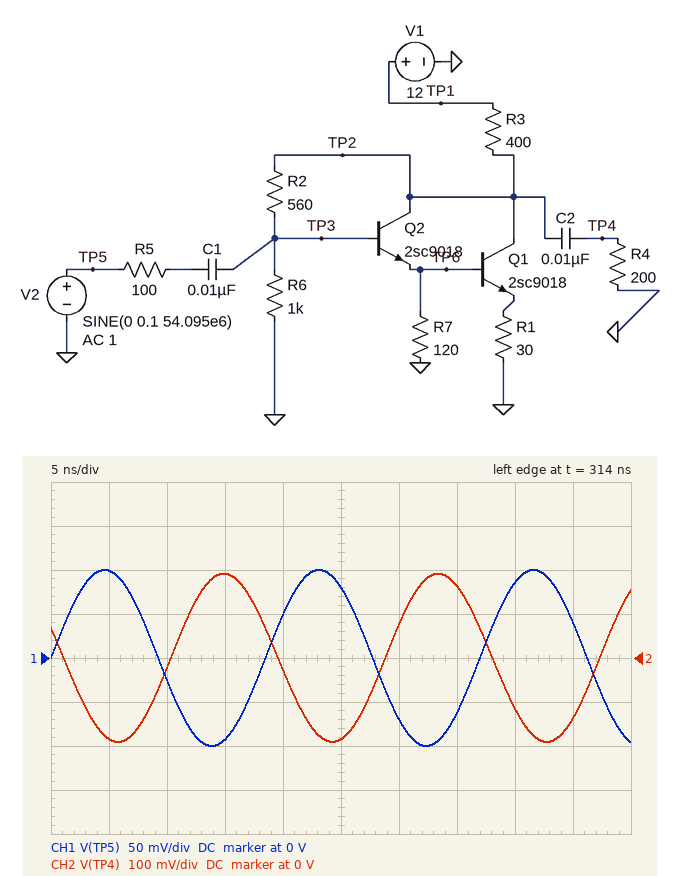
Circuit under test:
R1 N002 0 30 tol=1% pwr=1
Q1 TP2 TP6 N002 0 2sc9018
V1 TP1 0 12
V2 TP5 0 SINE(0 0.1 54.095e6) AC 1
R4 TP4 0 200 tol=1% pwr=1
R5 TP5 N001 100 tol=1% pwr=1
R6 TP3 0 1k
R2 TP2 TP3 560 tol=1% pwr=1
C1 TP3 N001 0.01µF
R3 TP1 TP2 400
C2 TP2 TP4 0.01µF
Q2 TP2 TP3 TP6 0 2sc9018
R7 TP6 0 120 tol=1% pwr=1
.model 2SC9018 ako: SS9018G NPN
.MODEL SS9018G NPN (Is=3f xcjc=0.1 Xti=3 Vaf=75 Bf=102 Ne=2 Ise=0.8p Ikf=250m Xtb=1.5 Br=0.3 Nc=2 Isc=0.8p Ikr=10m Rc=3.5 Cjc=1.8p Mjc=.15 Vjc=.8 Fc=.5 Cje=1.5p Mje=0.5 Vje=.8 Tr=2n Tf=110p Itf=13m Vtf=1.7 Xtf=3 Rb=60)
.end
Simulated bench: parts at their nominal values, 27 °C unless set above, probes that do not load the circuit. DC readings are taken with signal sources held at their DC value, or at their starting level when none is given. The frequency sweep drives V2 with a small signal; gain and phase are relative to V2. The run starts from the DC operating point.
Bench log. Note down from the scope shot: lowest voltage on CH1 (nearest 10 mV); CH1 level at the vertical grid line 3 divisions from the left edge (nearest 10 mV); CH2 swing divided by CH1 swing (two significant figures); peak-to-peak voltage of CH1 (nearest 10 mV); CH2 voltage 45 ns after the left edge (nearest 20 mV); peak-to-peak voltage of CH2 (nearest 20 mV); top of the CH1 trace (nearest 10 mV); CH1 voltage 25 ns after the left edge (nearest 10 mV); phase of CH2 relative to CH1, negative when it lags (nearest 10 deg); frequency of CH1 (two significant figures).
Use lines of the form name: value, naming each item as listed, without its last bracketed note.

lowest voltage on CH1: -100 mV
CH1 level at the vertical grid line 3 divisions from the left edge: -90 mV
CH2 swing divided by CH1 swing: 1.9
peak-to-peak voltage of CH1: 200 mV
CH2 voltage 45 ns after the left edge: -140 mV
peak-to-peak voltage of CH2: 380 mV
top of the CH1 trace: 100 mV
CH1 voltage 25 ns after the left edge: 80 mV
phase of CH2 relative to CH1, negative when it lags: 160 deg
frequency of CH1: 54 MHz
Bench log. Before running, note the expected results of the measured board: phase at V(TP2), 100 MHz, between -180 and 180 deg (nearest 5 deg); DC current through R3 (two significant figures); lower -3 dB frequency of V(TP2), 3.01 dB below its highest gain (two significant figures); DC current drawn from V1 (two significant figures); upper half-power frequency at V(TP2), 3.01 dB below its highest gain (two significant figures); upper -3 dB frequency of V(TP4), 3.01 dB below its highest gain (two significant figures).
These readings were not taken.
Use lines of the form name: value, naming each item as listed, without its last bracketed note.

phase at V(TP2), 100 MHz, between -180 and 180 deg: 140 deg
DC current through R3: 23 mA
lower -3 dB frequency of V(TP2), 3.01 dB below its highest gain: 55 kHz
DC current drawn from V1: 23 mA
upper half-power frequency at V(TP2), 3.01 dB below its highest gain: 220 MHz
upper -3 dB frequency of V(TP4), 3.01 dB below its highest gain: 220 MHz
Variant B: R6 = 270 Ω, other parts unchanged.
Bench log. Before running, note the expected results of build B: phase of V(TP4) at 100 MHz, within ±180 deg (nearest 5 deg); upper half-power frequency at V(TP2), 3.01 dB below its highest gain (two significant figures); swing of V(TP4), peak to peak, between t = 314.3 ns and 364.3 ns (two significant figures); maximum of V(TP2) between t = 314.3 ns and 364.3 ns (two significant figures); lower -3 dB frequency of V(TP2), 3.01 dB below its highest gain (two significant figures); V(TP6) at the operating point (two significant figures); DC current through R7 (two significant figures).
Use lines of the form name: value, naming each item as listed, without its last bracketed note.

phase of V(TP4) at 100 MHz, within ±180 deg: 150 deg
upper half-power frequency at V(TP2), 3.01 dB below its highest gain: 330 MHz
swing of V(TP4), peak to peak, between t = 314.3 ns and 364.3 ns: 320 mV
maximum of V(TP2) between t = 314.3 ns and 364.3 ns: 5.1 V
lower -3 dB frequency of V(TP2), 3.01 dB below its highest gain: 58 kHz
V(TP6) at the operating point: 860 mV
DC current through R7: 7.2 mA
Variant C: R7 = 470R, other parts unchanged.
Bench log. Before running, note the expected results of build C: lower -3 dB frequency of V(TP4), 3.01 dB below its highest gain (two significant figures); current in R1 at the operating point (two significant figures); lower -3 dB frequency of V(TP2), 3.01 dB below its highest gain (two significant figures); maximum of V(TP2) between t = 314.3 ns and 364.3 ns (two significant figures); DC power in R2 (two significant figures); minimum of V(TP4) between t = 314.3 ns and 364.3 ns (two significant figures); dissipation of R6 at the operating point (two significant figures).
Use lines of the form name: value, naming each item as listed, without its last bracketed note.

lower -3 dB frequency of V(TP4), 3.01 dB below its highest gain: 92 kHz
current in R1 at the operating point: 17 mA
lower -3 dB frequency of V(TP2), 3.01 dB below its highest gain: 50 kHz
maximum of V(TP2) between t = 314.3 ns and 364.3 ns: 3.3 V
DC power in R2: 2.3 mW
minimum of V(TP4) between t = 314.3 ns and 364.3 ns: -170 mV
dissipation of R6 at the operating point: 4.0 mW
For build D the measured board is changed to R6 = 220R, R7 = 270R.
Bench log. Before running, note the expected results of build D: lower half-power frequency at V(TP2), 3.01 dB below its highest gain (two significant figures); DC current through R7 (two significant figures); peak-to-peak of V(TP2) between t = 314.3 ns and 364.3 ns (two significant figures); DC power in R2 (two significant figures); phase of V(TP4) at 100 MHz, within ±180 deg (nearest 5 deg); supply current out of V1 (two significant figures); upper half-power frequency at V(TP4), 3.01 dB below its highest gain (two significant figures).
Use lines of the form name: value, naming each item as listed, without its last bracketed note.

lower half-power frequency at V(TP2), 3.01 dB below its highest gain: 56 kHz
DC current through R7: 3.3 mA
peak-to-peak of V(TP2) between t = 314.3 ns and 364.3 ns: 280 mV
DC power in R2: 30 mW
phase of V(TP4) at 100 MHz, within ±180 deg: 155 deg
supply current out of V1: 16 mA
upper half-power frequency at V(TP4), 3.01 dB below its highest gain: 380 MHz
